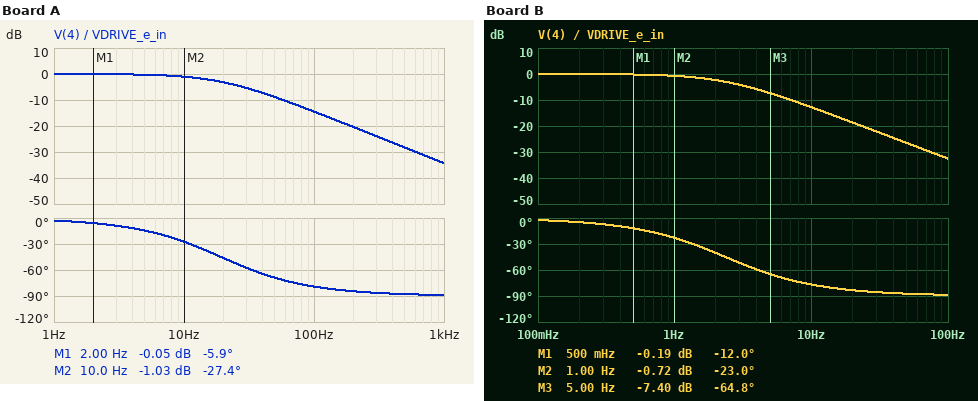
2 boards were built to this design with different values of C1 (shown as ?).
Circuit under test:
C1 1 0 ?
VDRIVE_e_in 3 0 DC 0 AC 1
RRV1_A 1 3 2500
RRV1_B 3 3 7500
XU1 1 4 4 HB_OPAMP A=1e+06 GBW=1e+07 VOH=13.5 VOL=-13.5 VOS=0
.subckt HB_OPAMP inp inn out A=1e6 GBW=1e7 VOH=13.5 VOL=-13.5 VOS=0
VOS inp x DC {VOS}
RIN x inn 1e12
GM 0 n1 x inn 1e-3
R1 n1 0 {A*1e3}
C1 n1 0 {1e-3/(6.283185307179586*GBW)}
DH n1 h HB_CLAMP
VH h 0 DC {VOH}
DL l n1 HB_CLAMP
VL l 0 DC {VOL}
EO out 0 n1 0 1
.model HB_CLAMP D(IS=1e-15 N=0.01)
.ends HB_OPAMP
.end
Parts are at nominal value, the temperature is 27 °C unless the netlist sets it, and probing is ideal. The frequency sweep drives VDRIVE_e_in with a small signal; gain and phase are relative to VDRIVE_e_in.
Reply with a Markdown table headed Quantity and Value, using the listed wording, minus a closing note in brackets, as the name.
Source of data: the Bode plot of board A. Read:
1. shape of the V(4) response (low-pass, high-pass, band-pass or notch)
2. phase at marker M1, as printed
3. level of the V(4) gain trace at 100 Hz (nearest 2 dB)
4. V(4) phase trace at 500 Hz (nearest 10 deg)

| Quantity | Value |
|---|---|
| shape of the V(4) response | low-pass |
| phase at marker M1, as printed | -5.9 deg |
| level of the V(4) gain trace at 100 Hz | -14 dB |
| V(4) phase trace at 500 Hz | -90 deg |
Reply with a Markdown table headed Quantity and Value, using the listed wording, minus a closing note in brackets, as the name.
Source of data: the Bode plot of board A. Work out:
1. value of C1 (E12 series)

| Quantity | Value |
|---|---|
| value of C1 | 3.3 µF |
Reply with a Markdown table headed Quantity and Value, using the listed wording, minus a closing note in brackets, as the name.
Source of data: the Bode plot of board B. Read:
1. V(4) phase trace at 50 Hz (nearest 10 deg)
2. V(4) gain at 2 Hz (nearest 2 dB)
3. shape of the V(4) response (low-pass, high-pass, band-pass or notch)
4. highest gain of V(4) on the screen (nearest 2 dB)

| Quantity | Value |
|---|---|
| V(4) phase trace at 50 Hz | -90 deg |
| V(4) gain at 2 Hz | -2 dB |
| shape of the V(4) response | low-pass |
| highest gain of V(4) on the screen | 0 dB |
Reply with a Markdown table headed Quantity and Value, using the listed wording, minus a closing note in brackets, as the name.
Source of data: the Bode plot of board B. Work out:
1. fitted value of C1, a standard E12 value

| Quantity | Value |
|---|---|
| fitted value of C1, a standard E12 value | 27 µF |
